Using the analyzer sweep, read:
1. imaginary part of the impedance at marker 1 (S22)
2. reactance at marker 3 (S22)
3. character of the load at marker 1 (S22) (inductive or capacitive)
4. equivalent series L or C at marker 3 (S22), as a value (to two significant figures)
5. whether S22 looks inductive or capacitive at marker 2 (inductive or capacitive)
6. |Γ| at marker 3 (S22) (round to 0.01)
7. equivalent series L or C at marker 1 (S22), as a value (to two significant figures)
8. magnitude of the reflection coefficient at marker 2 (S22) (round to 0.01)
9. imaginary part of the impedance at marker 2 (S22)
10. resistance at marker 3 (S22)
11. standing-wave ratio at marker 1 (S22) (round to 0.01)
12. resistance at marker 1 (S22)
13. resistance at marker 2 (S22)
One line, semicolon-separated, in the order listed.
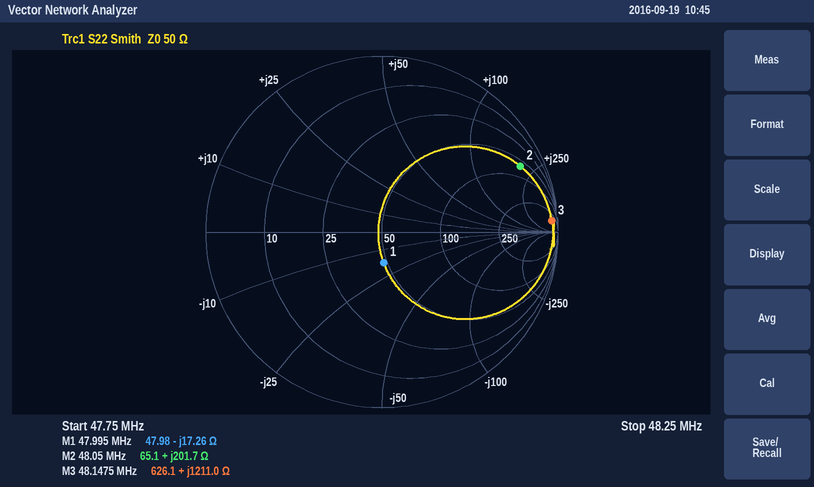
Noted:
-17.26 Ω; +1211.0 Ω; capacitive; 4.0 µH; inductive; 0.97; 190 pF; 0.87; +201.7 Ω; 626.1 Ω; 1.42; 47.98 Ω; 65.1 Ω
